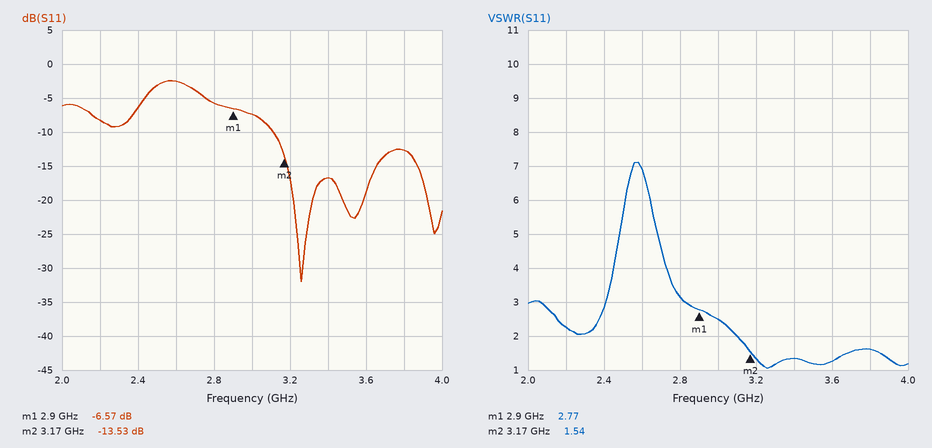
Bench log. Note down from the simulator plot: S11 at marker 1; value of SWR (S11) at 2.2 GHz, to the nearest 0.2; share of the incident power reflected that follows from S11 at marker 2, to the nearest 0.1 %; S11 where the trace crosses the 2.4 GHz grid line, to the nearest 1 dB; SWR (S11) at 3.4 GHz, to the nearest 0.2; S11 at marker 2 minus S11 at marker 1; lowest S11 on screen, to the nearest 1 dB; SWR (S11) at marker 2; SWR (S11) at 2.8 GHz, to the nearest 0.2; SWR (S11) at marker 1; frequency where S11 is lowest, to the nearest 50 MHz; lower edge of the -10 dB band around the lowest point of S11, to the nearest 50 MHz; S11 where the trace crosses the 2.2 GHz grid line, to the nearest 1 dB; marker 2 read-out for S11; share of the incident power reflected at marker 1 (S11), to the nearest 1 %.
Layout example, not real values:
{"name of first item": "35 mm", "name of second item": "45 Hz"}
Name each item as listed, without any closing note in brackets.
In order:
{"S11 at marker 1": "-6.57 dB", "value of SWR (S11) at 2.2 GHz, to the nearest 0.2": "2.2", "share of the incident power reflected that follows from S11 at marker 2, to the nearest 0.1 %": "4.4 %", "S11 where the trace crosses the 2.4 GHz grid line, to the nearest 1 dB": "-6 dB", "SWR (S11) at 3.4 GHz, to the nearest 0.2": "1.4", "S11 at marker 2 minus S11 at marker 1": "-6.96 dB", "lowest S11 on screen, to the nearest 1 dB": "-32 dB", "SWR (S11) at marker 2": "1.54", "SWR (S11) at 2.8 GHz, to the nearest 0.2": "3.2", "SWR (S11) at marker 1": "2.77", "frequency where S11 is lowest, to the nearest 50 MHz": "3.25 GHz", "lower edge of the -10 dB band around the lowest point of S11, to the nearest 50 MHz": "3.10 GHz", "S11 where the trace crosses the 2.2 GHz grid line, to the nearest 1 dB": "-8 dB", "marker 2 read-out for S11": "-13.53 dB", "share of the incident power reflected at marker 1 (S11), to the nearest 1 %": "22 %"}
